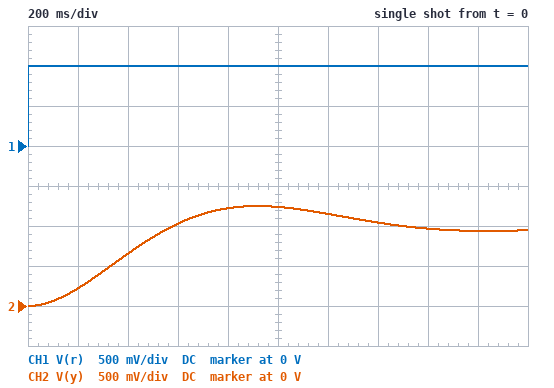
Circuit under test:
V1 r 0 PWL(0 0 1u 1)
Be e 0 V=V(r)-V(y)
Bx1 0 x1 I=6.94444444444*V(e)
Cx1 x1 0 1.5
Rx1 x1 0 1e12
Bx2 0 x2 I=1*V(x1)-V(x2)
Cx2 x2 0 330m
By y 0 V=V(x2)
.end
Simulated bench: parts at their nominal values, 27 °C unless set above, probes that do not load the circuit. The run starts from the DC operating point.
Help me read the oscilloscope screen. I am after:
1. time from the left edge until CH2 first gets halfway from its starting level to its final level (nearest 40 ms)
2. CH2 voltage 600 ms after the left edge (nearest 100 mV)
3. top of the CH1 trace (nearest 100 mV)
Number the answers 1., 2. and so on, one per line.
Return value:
1. 320 ms
2. 1.0 V
3. 1.0 V
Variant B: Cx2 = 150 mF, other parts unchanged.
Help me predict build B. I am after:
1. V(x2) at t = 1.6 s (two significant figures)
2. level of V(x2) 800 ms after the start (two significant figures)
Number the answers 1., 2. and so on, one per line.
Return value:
1. 990 mV
2. 1.1 V
